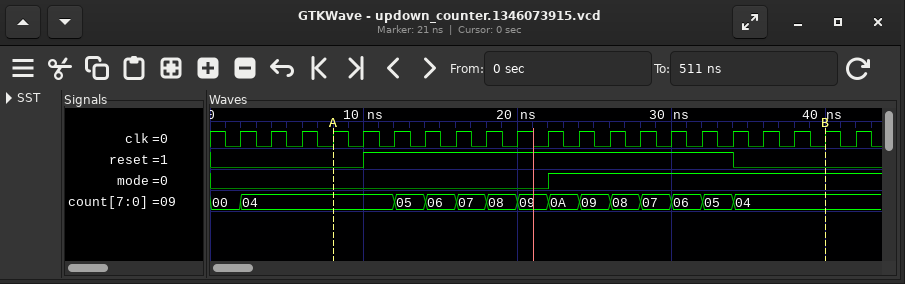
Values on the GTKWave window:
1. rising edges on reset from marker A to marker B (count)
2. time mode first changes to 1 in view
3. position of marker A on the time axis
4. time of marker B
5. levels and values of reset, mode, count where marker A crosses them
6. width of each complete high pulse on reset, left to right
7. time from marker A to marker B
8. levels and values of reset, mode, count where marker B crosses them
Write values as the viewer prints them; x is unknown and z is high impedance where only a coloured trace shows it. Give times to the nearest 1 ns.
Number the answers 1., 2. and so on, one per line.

1. 1
2. 22 ns
3. 8 ns
4. 40 ns
5. reset=0, mode=0, count=04
6. 24 ns
7. 32 ns
8. reset=0, mode=1, count=04
